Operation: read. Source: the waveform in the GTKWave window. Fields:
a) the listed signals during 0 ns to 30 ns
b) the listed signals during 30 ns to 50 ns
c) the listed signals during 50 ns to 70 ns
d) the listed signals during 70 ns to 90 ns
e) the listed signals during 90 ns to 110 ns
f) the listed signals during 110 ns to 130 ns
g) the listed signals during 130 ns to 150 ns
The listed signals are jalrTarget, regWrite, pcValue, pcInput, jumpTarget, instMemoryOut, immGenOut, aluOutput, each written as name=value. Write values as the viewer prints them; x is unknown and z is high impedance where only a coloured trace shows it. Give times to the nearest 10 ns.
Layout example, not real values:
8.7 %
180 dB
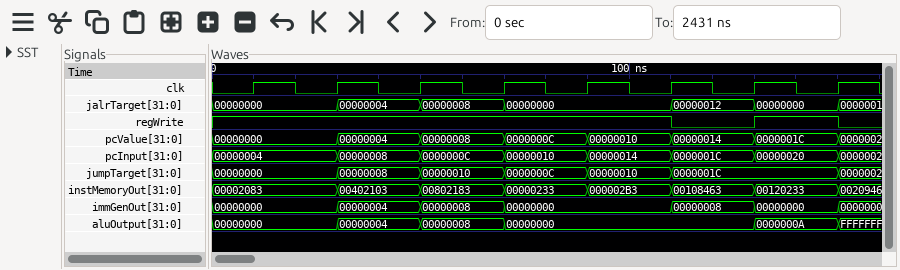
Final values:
jalrTarget=00000000, regWrite=1, pcValue=00000000, pcInput=00000004, jumpTarget=00000000, instMemoryOut=00002083, immGenOut=00000000, aluOutput=00000000
jalrTarget=00000004, regWrite=1, pcValue=00000004, pcInput=00000008, jumpTarget=00000008, instMemoryOut=00402103, immGenOut=00000004, aluOutput=00000004
jalrTarget=00000008, regWrite=1, pcValue=00000008, pcInput=0000000C, jumpTarget=00000010, instMemoryOut=00802183, immGenOut=00000008, aluOutput=00000008
jalrTarget=00000000, regWrite=1, pcValue=0000000C, pcInput=00000010, jumpTarget=0000000C, instMemoryOut=00000233, immGenOut=00000000, aluOutput=00000000
jalrTarget=00000000, regWrite=1, pcValue=00000010, pcInput=00000014, jumpTarget=00000010, instMemoryOut=000002B3, immGenOut=00000000, aluOutput=00000000
jalrTarget=00000012, regWrite=0, pcValue=00000014, pcInput=0000001C, jumpTarget=0000001C, instMemoryOut=00108463, immGenOut=00000008, aluOutput=00000000
jalrTarget=00000000, regWrite=1, pcValue=0000001C, pcInput=00000020, jumpTarget=0000001C, instMemoryOut=00120233, immGenOut=00000000, aluOutput=0000000A
